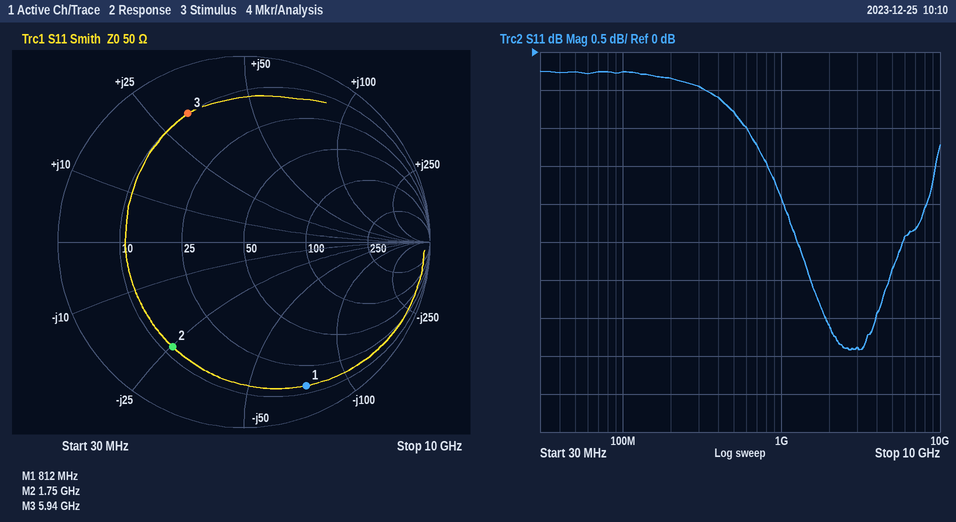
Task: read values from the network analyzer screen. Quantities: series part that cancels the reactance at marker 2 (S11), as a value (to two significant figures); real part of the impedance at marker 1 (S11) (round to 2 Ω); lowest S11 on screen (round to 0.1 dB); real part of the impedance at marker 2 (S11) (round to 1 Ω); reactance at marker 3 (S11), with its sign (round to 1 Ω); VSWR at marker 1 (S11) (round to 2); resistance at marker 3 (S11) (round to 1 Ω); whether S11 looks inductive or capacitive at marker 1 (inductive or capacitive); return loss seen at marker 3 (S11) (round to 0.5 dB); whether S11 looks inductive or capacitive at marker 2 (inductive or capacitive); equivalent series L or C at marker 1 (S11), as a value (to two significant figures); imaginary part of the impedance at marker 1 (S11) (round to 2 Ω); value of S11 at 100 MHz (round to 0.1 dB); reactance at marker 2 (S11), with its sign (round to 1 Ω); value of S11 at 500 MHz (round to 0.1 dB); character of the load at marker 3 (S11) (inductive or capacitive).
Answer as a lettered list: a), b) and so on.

a) 2.3 nH
b) 14 Ω
c) -3.9 dB
d) 12 Ω
e) +32 Ω
f) 12
g) 10 Ω
h) capacitive
i) 2.5 dB
j) capacitive
k) 2.6 pF
l) -74 Ω
m) -0.3 dB
n) -25 Ω
o) -0.8 dB
p) inductive
